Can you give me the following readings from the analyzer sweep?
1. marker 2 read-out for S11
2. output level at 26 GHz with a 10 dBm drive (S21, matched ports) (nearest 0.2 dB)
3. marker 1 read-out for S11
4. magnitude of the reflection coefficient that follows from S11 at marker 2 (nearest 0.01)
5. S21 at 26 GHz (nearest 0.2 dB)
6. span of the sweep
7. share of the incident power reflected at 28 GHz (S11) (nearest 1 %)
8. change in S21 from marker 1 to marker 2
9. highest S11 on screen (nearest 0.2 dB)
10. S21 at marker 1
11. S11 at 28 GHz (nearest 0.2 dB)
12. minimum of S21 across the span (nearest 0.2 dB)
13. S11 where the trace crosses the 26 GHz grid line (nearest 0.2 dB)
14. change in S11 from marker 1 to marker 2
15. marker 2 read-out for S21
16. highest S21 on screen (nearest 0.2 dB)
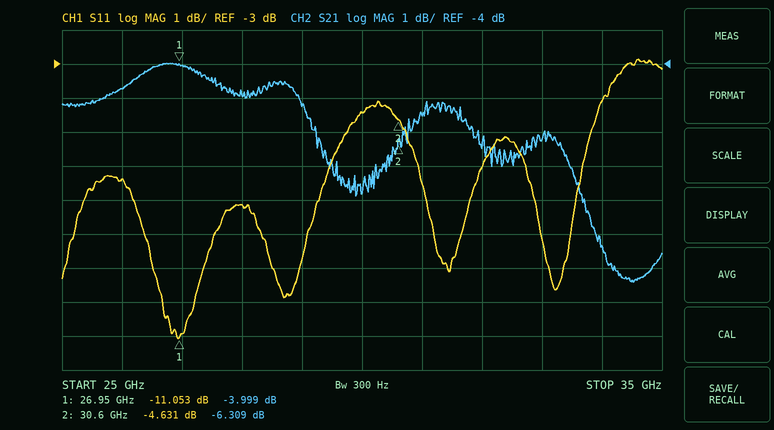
-4.631 dB
5.2 dBm
-11.053 dB
0.59
-4.8 dB
10 GHz
19 %
-2.310 dB
-2.8 dB
-3.999 dB
-7.2 dB
-10.4 dB
-6.4 dB
6.422 dB
-6.309 dB
-4.0 dB
